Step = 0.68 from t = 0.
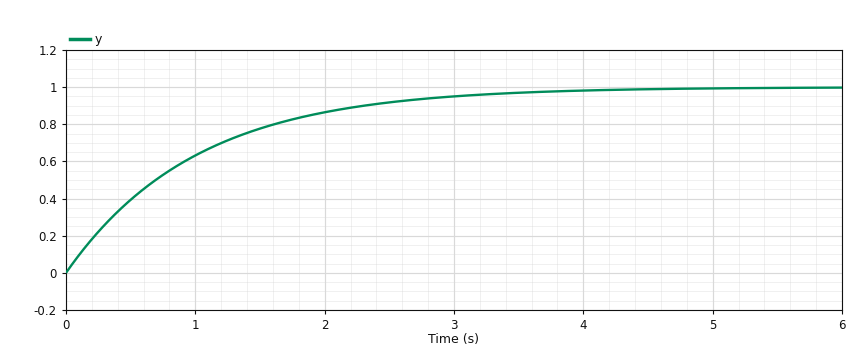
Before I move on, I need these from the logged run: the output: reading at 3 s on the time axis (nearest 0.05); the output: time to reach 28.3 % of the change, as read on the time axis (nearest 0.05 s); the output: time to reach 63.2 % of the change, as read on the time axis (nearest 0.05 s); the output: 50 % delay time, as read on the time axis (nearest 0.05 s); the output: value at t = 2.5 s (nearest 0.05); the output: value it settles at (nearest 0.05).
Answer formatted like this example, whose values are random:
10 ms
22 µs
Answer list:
0.95
0.35 s
1.00 s
0.70 s
0.90
1.00
